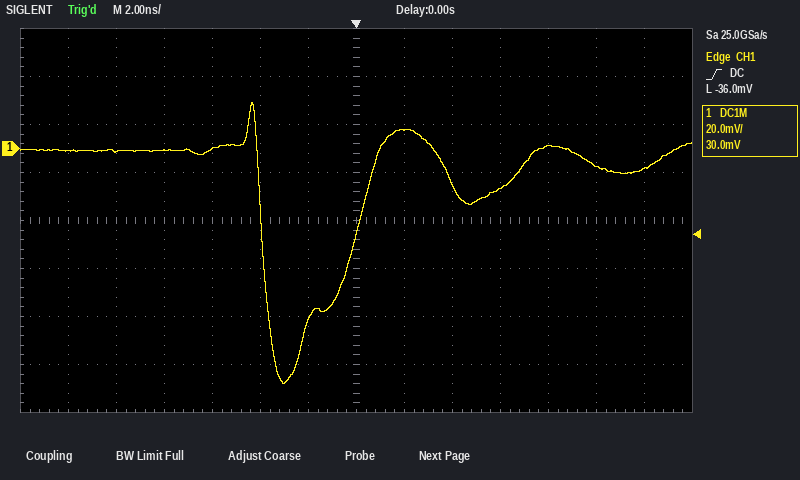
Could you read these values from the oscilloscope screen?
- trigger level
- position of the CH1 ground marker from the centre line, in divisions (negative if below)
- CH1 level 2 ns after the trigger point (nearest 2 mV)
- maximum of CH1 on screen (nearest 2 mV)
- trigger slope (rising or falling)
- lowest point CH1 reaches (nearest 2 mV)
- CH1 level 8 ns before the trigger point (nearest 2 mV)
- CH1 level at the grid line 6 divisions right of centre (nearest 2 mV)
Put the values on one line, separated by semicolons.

-36.0 mV; +1.5 div; 8 mV; 20 mV; rising; -98 mV; 0 mV; -8 mV
